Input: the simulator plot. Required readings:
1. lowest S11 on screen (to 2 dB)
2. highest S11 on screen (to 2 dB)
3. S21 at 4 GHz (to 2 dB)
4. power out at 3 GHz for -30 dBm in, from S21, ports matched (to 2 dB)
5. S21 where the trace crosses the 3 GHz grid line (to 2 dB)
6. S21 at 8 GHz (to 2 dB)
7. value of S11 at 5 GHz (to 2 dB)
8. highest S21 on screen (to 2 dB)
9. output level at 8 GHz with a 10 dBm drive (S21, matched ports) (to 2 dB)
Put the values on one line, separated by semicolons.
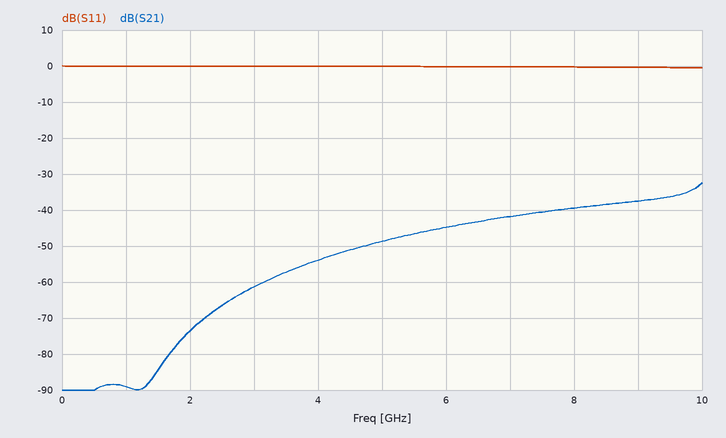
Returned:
0 dB; 0 dB; -54 dB; -92 dBm; -62 dB; -40 dB; 0 dB; -32 dB; -30 dBm
